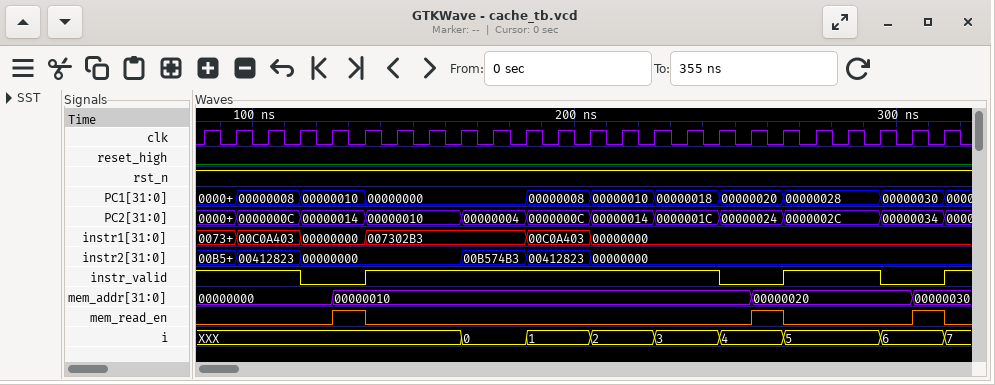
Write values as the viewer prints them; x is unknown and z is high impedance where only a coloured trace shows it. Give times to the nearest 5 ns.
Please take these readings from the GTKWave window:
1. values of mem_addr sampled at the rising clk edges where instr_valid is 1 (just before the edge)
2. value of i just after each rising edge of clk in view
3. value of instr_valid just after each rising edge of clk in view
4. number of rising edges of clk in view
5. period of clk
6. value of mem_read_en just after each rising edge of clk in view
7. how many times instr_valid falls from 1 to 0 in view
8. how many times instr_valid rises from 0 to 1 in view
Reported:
00000000, 00000000, 00000000, 00000000, 00000010, 00000010, 00000010, 00000010, 00000010, 00000010, 00000010, 00000010, 00000010, 00000010, 00000010, 00000020, 00000020, 00000020
XXX, XXX, XXX, XXX, XXX, XXX, XXX, XXX, 0, 0, 1, 1, 2, 2, 3, 3, 4, 4, 5, 5, 5, 6, 6, 7
1 1 1 0 0 1 1 1 1 1 1 1 1 1 1 1 0 0 1 1 1 0 0 1
24
10 ns
0 0 0 0 1 0 0 0 0 0 0 0 0 0 0 0 0 1 0 0 0 0 1 0
3
3
